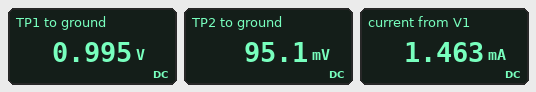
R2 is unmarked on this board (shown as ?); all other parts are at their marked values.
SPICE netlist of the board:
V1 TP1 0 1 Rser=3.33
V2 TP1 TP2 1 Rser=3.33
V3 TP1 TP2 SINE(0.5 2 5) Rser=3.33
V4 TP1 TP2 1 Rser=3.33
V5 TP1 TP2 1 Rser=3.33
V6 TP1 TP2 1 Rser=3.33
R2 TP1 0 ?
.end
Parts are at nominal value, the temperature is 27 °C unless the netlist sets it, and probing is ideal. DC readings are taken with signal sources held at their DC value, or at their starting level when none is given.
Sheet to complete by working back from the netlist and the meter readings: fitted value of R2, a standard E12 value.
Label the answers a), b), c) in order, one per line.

a) 680 Ω
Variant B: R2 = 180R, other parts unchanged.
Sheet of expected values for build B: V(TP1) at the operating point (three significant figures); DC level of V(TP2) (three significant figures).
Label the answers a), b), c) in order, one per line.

a) 982 mV
b) 81.8 mV
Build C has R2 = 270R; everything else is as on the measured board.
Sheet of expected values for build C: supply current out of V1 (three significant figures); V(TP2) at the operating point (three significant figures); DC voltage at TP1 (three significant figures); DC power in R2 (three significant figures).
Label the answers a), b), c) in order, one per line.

a) 3.66 mA
b) 87.8 mV
c) 988 mV
d) 3.61 mW
